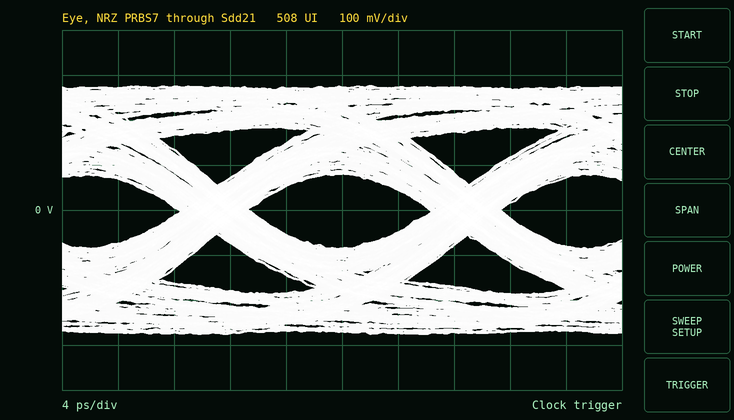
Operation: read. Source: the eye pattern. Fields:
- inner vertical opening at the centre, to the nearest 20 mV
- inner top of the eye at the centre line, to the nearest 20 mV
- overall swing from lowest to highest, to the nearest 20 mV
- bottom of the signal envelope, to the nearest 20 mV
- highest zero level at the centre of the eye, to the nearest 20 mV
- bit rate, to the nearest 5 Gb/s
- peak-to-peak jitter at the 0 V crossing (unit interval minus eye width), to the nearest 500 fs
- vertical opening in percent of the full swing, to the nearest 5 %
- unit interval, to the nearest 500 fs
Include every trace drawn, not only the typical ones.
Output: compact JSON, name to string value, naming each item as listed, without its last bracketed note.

{"inner vertical opening at the centre, to the nearest 20 mV": "160 mV", "inner top of the eye at the centre line, to the nearest 20 mV": "80 mV", "overall swing from lowest to highest, to the nearest 20 mV": "560 mV", "bottom of the signal envelope, to the nearest 20 mV": "-280 mV", "highest zero level at the centre of the eye, to the nearest 20 mV": "-80 mV", "bit rate, to the nearest 5 Gb/s": "55 Gb/s", "peak-to-peak jitter at the 0 V crossing (unit interval minus eye width), to the nearest 500 fs": "5.0 ps", "vertical opening in percent of the full swing, to the nearest 5 %": "30 %", "unit interval, to the nearest 500 fs": "18.0 ps"}
